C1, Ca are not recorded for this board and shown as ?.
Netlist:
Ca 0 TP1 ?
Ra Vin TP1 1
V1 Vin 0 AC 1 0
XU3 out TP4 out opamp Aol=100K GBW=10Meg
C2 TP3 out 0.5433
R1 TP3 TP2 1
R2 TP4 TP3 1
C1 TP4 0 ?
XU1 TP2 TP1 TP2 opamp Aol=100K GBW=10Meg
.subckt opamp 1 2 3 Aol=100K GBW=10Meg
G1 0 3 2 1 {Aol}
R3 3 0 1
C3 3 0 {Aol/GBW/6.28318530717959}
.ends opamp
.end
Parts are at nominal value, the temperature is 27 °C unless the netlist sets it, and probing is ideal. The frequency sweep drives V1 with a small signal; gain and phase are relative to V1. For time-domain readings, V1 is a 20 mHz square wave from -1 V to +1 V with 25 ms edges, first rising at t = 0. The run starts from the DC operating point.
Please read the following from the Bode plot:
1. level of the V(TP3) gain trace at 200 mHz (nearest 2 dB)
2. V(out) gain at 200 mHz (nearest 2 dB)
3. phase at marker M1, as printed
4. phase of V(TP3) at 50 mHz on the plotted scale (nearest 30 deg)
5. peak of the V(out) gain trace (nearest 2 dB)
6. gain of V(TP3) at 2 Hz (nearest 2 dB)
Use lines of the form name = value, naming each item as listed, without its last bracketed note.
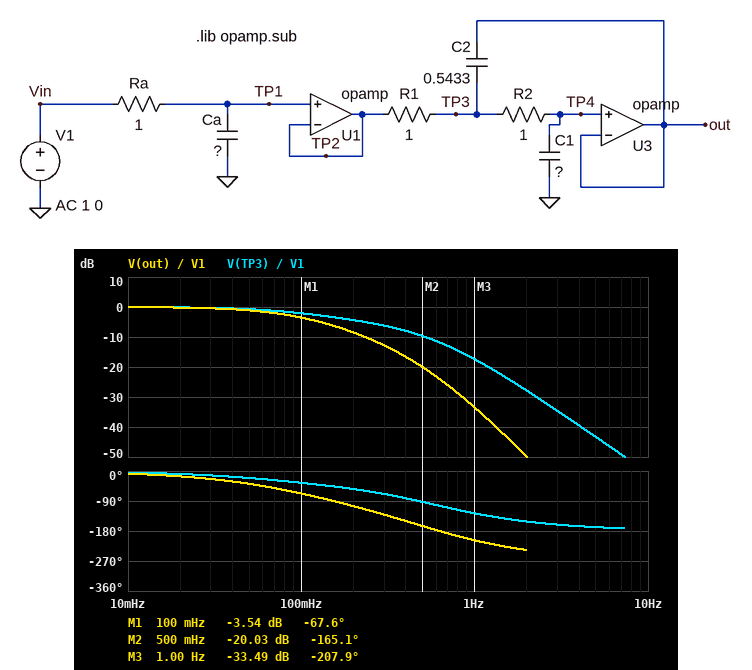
level of the V(TP3) gain trace at 200 mHz = -4 dB
V(out) gain at 200 mHz = -8 dB
phase at marker M1, as printed = -67.6 deg
phase of V(TP3) at 50 mHz on the plotted scale = -30 deg
peak of the V(out) gain trace = 0 dB
gain of V(TP3) at 2 Hz = -28 dB
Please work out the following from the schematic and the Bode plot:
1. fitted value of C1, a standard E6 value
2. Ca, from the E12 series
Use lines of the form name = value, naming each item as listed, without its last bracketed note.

fitted value of C1, a standard E6 value = 1 F
Ca, from the E12 series = 270 mF
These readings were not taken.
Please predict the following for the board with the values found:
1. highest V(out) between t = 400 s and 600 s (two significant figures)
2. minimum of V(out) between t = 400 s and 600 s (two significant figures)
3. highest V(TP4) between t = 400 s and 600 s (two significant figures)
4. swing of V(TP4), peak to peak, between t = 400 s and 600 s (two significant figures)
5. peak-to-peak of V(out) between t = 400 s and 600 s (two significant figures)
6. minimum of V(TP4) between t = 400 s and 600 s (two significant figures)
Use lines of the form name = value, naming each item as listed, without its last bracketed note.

highest V(out) between t = 400 s and 600 s = 1.0 V
minimum of V(out) between t = 400 s and 600 s = -1.0 V
highest V(TP4) between t = 400 s and 600 s = 1.0 V
swing of V(TP4), peak to peak, between t = 400 s and 600 s = 2.0 V
peak-to-peak of V(out) between t = 400 s and 600 s = 2.0 V
minimum of V(TP4) between t = 400 s and 600 s = -1.0 V
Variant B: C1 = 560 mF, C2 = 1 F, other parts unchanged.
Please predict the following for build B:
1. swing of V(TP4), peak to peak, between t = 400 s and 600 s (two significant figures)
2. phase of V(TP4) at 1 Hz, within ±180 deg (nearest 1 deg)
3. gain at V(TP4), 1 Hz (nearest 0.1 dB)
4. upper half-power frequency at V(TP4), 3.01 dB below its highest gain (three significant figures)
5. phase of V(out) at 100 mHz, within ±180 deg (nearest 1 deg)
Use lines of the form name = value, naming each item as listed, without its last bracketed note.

swing of V(TP4), peak to peak, between t = 400 s and 600 s = 2.1 V
phase of V(TP4) at 1 Hz, within ±180 deg = 139 deg
gain at V(TP4), 1 Hz = -32.8 dB
upper half-power frequency at V(TP4), 3.01 dB below its highest gain = 189 mHz
phase of V(out) at 100 mHz, within ±180 deg = -52 deg
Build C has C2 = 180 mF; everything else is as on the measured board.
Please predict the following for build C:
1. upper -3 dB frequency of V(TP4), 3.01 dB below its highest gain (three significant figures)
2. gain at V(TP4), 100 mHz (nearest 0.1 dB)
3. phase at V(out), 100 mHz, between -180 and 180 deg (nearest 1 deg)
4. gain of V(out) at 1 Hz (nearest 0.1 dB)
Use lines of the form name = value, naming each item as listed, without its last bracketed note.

upper -3 dB frequency of V(TP4), 3.01 dB below its highest gain = 81.7 mHz
gain at V(TP4), 100 mHz = -4.0 dB
phase at V(out), 100 mHz, between -180 and 180 deg = -63 deg
gain of V(out) at 1 Hz = -28.8 dB
